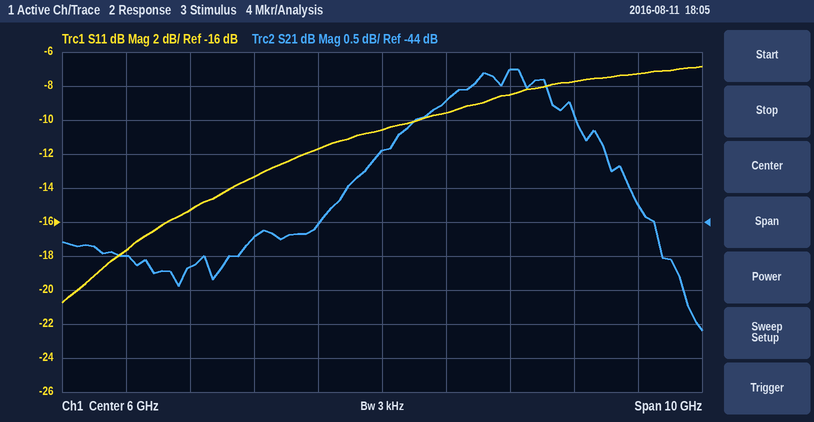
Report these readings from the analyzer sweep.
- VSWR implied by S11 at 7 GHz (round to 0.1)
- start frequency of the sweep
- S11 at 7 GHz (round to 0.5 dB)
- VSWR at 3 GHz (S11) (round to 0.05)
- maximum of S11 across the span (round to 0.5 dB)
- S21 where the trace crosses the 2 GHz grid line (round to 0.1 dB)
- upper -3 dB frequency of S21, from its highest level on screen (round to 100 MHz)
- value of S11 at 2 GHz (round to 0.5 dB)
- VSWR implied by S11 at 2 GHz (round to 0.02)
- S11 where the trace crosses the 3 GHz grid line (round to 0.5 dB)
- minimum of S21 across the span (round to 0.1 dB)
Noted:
2.0
1 GHz
-9.5 dB
1.40
-7.0 dB
-44.5 dB
10.6 GHz
-17.5 dB
1.30
-15.5 dB
-45.6 dB
